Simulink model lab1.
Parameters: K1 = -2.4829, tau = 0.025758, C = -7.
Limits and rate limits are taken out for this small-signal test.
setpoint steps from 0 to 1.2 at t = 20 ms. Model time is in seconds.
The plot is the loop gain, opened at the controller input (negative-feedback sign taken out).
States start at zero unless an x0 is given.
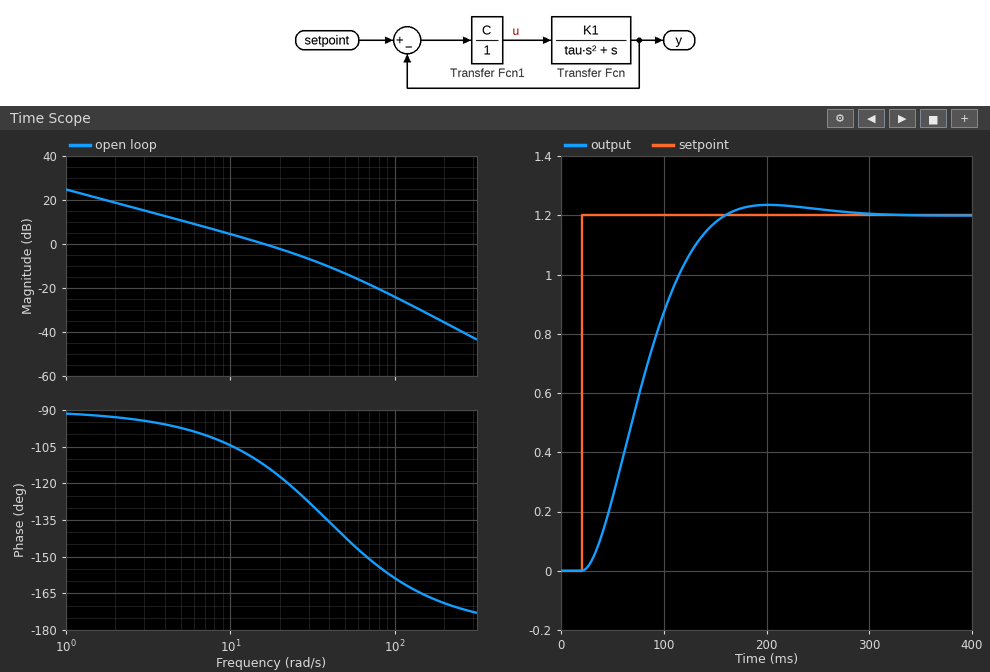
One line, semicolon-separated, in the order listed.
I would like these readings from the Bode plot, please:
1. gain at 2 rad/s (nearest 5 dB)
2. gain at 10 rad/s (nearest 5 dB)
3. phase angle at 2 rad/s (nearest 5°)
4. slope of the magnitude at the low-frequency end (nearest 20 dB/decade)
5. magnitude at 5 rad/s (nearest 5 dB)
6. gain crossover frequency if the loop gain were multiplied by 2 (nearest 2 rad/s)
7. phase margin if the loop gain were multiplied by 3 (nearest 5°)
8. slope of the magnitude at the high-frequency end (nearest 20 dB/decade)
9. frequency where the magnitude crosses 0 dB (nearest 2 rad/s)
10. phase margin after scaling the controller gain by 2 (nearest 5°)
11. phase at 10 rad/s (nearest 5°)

20 dB; 5 dB; -95°; -20 dB/decade; 10 dB; 28 rad/s; 45°; -40 dB/decade; 16 rad/s; 55°; -105°
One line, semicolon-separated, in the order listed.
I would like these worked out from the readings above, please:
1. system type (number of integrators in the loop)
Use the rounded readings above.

1
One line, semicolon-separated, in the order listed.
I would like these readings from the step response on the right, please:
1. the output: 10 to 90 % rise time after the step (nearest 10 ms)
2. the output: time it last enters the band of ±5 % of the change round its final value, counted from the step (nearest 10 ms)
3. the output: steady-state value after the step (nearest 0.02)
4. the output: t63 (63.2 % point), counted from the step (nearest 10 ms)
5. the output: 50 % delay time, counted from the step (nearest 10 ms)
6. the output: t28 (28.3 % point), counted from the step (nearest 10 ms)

90 ms; 120 ms; 1.20; 70 ms; 60 ms; 40 ms
